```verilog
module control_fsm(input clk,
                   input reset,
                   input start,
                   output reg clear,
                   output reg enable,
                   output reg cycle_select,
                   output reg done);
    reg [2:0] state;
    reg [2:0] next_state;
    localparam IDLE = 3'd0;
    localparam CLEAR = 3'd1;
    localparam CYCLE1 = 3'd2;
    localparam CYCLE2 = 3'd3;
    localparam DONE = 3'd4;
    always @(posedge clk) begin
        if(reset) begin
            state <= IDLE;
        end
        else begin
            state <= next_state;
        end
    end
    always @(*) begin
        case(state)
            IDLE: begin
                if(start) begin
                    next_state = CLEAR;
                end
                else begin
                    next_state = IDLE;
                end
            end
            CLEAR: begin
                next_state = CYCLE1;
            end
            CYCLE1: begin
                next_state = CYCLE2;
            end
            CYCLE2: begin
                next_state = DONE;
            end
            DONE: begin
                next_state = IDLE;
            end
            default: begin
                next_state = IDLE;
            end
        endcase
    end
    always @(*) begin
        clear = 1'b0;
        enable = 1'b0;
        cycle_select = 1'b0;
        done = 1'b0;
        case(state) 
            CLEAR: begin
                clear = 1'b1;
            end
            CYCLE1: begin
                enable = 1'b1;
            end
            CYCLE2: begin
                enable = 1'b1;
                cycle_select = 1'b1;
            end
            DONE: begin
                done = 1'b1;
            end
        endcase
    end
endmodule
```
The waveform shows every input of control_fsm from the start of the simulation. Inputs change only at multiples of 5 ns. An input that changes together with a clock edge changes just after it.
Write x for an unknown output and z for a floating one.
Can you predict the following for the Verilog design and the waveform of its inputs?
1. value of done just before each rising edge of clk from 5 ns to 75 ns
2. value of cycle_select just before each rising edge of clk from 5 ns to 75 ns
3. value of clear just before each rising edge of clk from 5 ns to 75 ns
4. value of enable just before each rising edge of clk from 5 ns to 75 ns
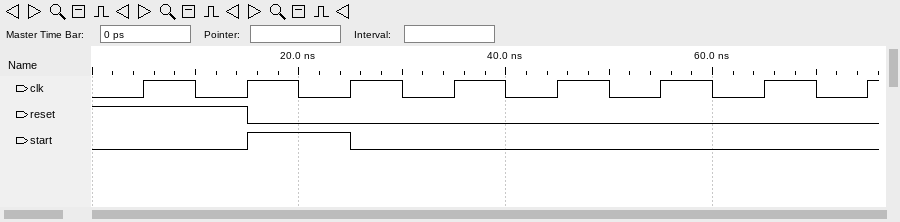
x 0 0 0 0 0 1 0
x 0 0 0 0 1 0 0
x 0 0 1 0 0 0 0
x 0 0 0 1 1 0 0
